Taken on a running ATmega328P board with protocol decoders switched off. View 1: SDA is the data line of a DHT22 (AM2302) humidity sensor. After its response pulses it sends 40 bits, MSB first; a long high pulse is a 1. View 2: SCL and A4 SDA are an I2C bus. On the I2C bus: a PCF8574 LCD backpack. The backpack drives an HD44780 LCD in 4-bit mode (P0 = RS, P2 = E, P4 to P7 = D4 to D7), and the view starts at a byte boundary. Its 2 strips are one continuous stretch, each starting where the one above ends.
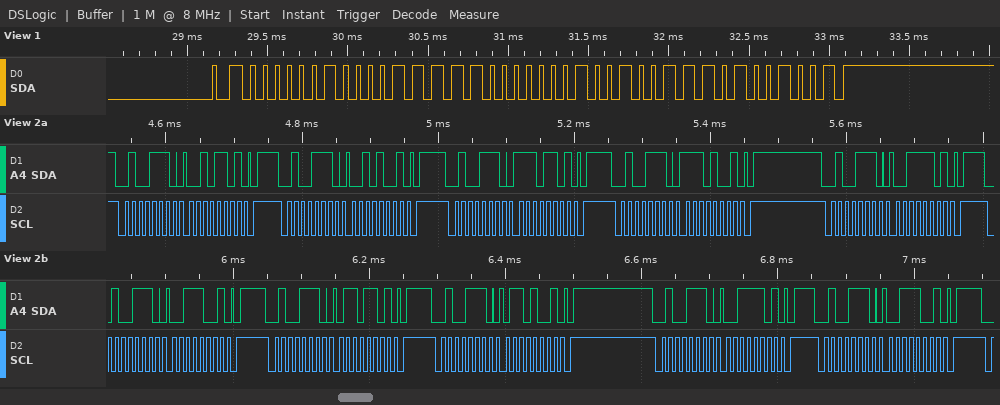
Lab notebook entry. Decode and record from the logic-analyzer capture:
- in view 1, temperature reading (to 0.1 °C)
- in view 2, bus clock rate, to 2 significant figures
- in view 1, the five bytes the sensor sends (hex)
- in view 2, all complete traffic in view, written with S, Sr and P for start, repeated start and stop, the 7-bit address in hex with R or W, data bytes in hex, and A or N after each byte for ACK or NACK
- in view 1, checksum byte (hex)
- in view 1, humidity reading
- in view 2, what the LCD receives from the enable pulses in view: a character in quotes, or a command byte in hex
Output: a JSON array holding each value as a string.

["29.5 °C", "100 kHz", "02 1F 01 27 49", "S 27W A 2D A P S 27W A 29 A P S 27W A ED A P S 27W A E9 A P S 27W A 3D A P S 27W A 39 A P S 27W A 6D A P S 27W A 69 A P S 27W A 3D A P S 27W A 39 A P", "0x49", "54.3 %", "'.' '6'"]
